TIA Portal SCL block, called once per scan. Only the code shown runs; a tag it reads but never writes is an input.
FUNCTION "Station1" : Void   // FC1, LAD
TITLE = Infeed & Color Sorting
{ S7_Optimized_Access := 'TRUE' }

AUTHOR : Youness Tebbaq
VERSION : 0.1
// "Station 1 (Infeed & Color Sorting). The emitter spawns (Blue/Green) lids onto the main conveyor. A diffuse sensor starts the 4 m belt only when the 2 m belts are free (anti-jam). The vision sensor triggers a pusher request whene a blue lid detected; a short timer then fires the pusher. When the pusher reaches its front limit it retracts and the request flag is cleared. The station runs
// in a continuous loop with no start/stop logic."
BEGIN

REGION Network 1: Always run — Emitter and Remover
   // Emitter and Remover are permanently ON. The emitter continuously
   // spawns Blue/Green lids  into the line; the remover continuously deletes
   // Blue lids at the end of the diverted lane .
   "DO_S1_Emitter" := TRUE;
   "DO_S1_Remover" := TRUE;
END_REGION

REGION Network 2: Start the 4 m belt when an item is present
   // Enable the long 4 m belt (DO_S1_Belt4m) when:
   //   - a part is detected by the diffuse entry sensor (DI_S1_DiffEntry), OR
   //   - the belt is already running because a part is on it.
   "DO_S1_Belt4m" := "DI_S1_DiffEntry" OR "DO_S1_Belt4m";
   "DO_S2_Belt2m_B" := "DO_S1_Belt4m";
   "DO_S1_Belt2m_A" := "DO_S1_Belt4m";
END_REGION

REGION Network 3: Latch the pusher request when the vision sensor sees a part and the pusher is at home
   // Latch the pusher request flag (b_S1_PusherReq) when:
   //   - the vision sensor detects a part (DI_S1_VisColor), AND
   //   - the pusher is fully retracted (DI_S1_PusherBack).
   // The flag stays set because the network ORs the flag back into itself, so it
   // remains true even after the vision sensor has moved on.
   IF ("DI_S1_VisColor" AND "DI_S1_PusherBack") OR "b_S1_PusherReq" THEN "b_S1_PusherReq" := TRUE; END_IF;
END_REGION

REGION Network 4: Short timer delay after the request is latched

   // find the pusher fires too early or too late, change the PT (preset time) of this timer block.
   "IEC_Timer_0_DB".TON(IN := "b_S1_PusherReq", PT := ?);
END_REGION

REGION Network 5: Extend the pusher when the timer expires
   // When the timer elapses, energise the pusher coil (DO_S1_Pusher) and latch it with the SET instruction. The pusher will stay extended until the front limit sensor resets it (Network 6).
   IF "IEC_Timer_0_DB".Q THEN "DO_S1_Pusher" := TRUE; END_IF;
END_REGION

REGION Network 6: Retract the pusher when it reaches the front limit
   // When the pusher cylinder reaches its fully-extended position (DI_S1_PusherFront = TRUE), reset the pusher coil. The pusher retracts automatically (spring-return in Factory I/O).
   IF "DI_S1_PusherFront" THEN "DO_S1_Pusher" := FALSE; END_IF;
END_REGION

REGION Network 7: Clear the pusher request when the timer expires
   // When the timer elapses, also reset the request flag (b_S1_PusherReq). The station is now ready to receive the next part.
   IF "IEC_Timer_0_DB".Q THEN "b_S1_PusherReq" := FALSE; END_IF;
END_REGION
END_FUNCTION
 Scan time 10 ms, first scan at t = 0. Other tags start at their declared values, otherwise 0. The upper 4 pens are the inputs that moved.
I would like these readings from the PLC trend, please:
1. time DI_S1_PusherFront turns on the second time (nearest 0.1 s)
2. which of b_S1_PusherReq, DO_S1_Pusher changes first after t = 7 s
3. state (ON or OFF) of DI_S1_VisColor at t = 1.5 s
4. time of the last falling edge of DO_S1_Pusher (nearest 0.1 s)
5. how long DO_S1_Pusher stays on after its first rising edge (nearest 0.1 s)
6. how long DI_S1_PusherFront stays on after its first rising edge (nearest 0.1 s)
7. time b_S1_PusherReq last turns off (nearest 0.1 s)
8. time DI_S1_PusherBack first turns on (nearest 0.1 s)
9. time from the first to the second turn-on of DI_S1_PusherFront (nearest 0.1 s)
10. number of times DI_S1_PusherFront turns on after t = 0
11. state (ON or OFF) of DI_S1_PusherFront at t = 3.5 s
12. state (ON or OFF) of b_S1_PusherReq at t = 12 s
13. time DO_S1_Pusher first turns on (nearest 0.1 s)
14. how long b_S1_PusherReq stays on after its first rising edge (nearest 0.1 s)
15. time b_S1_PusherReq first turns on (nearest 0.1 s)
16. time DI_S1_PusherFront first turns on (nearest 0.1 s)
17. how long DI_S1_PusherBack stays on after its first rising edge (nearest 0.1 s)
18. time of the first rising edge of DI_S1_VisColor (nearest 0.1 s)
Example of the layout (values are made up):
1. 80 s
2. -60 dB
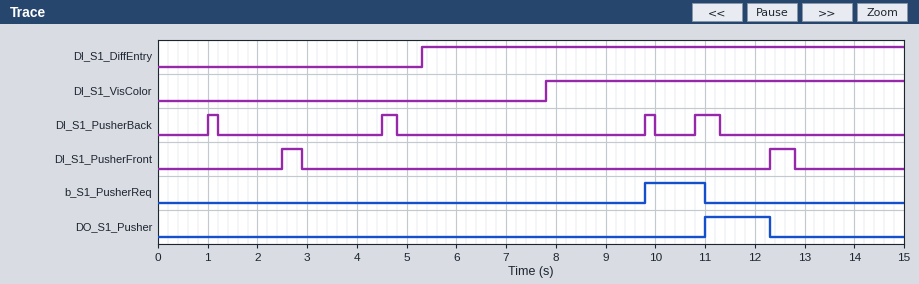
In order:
1. 12.3 s
2. b_S1_PusherReq
3. OFF
4. 12.3 s
5. 1.3 s
6. 0.4 s
7. 11.0 s
8. 1.0 s
9. 9.8 s
10. 2
11. OFF
12. OFF
13. 11.0 s
14. 1.2 s
15. 9.8 s
16. 2.5 s
17. 0.2 s
18. 7.8 s
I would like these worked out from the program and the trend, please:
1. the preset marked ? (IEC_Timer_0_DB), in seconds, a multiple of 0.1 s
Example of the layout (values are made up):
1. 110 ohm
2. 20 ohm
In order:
1. 1.2 s
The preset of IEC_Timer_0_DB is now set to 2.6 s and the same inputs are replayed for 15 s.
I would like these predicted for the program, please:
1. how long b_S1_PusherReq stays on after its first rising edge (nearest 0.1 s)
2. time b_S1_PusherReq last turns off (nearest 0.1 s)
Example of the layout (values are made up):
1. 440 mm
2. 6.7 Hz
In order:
1. 2.6 s
2. 12.4 s
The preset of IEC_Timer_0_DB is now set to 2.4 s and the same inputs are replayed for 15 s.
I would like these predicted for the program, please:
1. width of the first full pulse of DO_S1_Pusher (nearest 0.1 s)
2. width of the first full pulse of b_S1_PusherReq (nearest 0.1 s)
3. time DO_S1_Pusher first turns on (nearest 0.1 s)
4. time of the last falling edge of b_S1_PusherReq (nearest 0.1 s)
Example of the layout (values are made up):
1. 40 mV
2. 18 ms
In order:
1. 0.1 s
2. 2.4 s
3. 12.2 s
4. 12.2 s
